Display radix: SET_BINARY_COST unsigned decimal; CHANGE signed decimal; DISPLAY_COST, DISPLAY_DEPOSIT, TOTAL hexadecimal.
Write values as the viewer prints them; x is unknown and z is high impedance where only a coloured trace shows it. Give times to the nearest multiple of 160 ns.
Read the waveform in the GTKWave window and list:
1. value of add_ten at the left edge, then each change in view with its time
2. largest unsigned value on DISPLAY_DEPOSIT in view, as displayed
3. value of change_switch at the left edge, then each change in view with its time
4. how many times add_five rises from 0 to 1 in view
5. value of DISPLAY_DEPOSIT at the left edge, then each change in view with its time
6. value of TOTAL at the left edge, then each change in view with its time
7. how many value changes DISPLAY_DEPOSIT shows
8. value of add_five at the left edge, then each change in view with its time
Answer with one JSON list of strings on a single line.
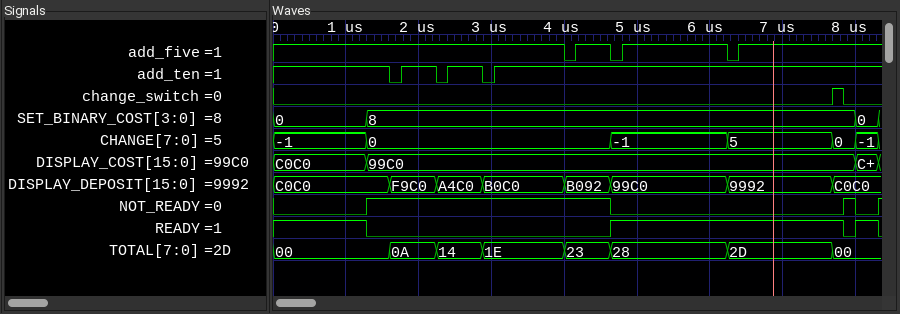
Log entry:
["1, 0 at 1600 ns, 1 at 1760 ns, 0 at 2240 ns, 1 at 2400 ns, 0 at 2880 ns, 1 at 3040 ns", "F9C0", "0, 1 at 7680 ns, 0 at 7840 ns", "3", "C0C0, F9C0 at 1600 ns, A4C0 at 2240 ns, B0C0 at 2880 ns, B092 at 4000 ns, 99C0 at 4640 ns, 9992 at 6240 ns, C0C0 at 7680 ns", "00, 0A at 1600 ns, 14 at 2240 ns, 1E at 2880 ns, 23 at 4000 ns, 28 at 4640 ns, 2D at 6240 ns, 00 at 7680 ns", "7", "1, 0 at 4000 ns, 1 at 4160 ns, 0 at 4640 ns, 1 at 4800 ns, 0 at 6240 ns, 1 at 6400 ns"]
